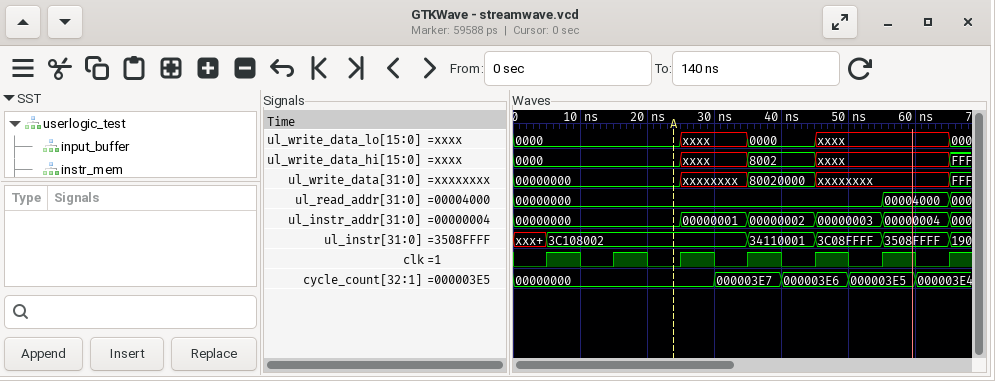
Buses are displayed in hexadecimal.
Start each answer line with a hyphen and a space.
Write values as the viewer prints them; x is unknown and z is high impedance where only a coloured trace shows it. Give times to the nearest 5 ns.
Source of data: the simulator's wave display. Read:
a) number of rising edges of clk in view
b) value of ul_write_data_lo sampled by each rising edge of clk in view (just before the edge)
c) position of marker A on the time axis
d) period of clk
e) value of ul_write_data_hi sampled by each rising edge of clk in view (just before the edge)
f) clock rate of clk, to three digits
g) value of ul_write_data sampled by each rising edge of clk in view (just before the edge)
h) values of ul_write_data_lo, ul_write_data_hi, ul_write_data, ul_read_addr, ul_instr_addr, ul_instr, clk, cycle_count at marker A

- 7
- 0000, 0000, 0000, xxxx, 0000, xxxx, xxxx
- 25 ns
- 10 ns
- 0000, 0000, 0000, xxxx, 8002, xxxx, xxxx
- 100 MHz
- 00000000, 00000000, 00000000, xxxxxxxx, 80020000, xxxxxxxx, xxxxxxxx
- ul_write_data_lo=0000, ul_write_data_hi=0000, ul_write_data=00000000, ul_read_addr=00000000, ul_instr_addr=00000000, ul_instr=3C108002, clk=0, cycle_count=00000000
